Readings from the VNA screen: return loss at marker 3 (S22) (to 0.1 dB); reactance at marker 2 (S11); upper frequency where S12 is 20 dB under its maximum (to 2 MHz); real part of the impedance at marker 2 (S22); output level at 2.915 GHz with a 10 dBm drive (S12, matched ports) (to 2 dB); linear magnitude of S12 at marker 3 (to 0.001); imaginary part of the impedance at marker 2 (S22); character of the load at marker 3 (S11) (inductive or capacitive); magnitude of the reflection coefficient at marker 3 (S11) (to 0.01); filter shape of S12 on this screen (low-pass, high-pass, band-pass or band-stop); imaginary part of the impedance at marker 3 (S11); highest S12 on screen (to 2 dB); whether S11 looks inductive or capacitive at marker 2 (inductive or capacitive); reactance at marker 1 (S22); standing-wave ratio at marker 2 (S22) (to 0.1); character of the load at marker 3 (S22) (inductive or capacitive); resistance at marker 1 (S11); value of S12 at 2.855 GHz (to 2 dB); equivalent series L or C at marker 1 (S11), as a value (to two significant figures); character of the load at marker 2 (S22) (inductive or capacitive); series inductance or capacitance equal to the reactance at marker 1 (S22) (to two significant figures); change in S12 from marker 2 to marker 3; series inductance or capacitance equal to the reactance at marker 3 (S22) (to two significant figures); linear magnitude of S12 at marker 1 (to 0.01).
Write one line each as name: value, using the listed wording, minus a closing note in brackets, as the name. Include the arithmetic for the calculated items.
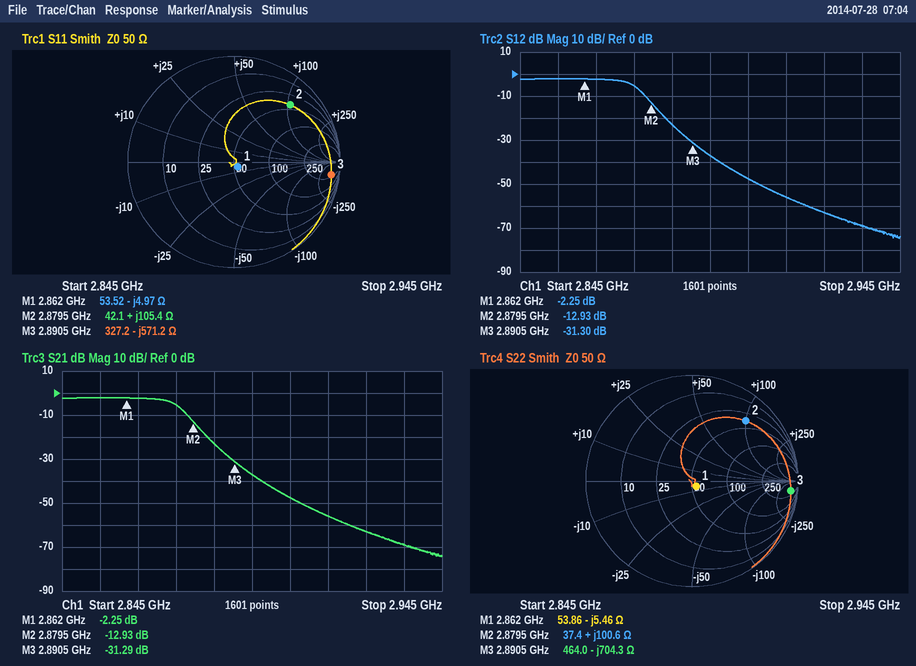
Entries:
return loss at marker 3 (S22): 0.6 dB
reactance at marker 2: +105.4 Ω
upper frequency where S12 is 20 dB under its maximum: 2.884 GHz
real part of the impedance at marker 2: 37.4 Ω
output level at 2.915 GHz with a 10 dBm drive (S12, matched ports): 10 dBm + (-56 dB) = -46 dBm
linear magnitude of S12 at marker 3: 10^(-31.3/20) ≈ 0.027
imaginary part of the impedance at marker 2: +100.6 Ω
character of the load at marker 3 (S11): capacitive
magnitude of the reflection coefficient at marker 3 (S11): 0.93
filter shape of S12 on this screen: low-pass
imaginary part of the impedance at marker 3: -571.2 Ω
highest S12 on screen: -2 dB
whether S11 looks inductive or capacitive at marker 2: inductive
reactance at marker 1: -5.46 Ω
standing-wave ratio at marker 2 (S22): 7.4
character of the load at marker 3 (S22): capacitive
resistance at marker 1: 53.52 Ω
value of S12 at 2.855 GHz: -2 dB
equivalent series L or C at marker 1 (S11), as a value: C = 1/(2π × 2.862 GHz × 4.97 Ω) ≈ 11 pF
character of the load at marker 2 (S22): inductive
series inductance or capacitance equal to the reactance at marker 1 (S22): C = 1/(2π × 2.862 GHz × 5.46 Ω) ≈ 10 pF
change in S12 from marker 2 to marker 3: -31.3 − (-12.93) = -18.37 dB
series inductance or capacitance equal to the reactance at marker 3 (S22): C = 1/(2π × 2.8905 GHz × 704.3 Ω) ≈ 78 fF
linear magnitude of S12 at marker 1: 10^(-2.25/20) ≈ 0.77
